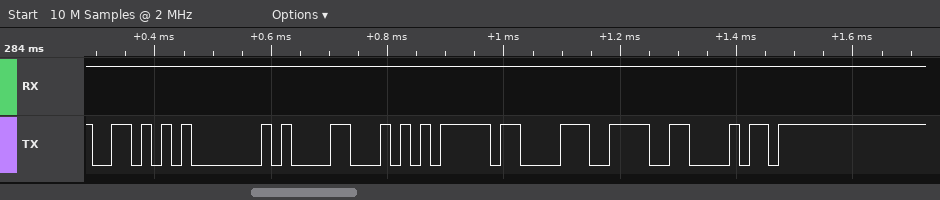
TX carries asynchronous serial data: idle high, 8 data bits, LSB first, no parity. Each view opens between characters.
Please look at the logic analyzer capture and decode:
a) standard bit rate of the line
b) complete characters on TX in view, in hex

57600 baud
56, 40, 18, F5, C3, 9E, 68
